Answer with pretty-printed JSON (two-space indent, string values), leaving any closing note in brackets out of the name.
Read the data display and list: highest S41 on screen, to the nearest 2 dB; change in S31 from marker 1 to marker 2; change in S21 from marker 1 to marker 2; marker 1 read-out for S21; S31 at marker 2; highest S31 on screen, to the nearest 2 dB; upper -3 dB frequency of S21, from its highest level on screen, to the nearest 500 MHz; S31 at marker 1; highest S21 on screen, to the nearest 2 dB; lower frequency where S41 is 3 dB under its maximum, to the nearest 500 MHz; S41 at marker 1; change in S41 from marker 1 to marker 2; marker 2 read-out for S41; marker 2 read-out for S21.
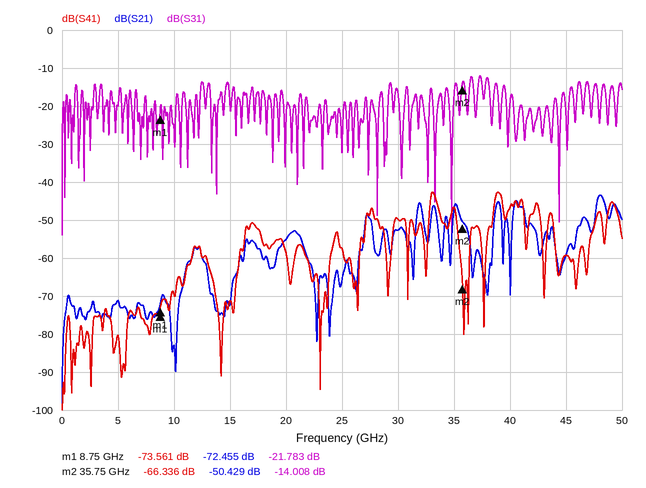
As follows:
{
  "highest S41 on screen, to the nearest 2 dB": "-42 dB",
  "change in S31 from marker 1 to marker 2": "7.775 dB",
  "change in S21 from marker 1 to marker 2": "22.026 dB",
  "marker 1 read-out for S21": "-72.455 dB",
  "S31 at marker 2": "-14.008 dB",
  "highest S31 on screen, to the nearest 2 dB": "-12 dB",
  "upper -3 dB frequency of S21, from its highest level on screen, to the nearest 500 MHz": "48.5 GHz",
  "S31 at marker 1": "-21.783 dB",
  "highest S21 on screen, to the nearest 2 dB": "-44 dB",
  "lower frequency where S41 is 3 dB under its maximum, to the nearest 500 MHz": "33.0 GHz",
  "S41 at marker 1": "-73.561 dB",
  "change in S41 from marker 1 to marker 2": "7.225 dB",
  "marker 2 read-out for S41": "-66.336 dB",
  "marker 2 read-out for S21": "-50.429 dB"
}
